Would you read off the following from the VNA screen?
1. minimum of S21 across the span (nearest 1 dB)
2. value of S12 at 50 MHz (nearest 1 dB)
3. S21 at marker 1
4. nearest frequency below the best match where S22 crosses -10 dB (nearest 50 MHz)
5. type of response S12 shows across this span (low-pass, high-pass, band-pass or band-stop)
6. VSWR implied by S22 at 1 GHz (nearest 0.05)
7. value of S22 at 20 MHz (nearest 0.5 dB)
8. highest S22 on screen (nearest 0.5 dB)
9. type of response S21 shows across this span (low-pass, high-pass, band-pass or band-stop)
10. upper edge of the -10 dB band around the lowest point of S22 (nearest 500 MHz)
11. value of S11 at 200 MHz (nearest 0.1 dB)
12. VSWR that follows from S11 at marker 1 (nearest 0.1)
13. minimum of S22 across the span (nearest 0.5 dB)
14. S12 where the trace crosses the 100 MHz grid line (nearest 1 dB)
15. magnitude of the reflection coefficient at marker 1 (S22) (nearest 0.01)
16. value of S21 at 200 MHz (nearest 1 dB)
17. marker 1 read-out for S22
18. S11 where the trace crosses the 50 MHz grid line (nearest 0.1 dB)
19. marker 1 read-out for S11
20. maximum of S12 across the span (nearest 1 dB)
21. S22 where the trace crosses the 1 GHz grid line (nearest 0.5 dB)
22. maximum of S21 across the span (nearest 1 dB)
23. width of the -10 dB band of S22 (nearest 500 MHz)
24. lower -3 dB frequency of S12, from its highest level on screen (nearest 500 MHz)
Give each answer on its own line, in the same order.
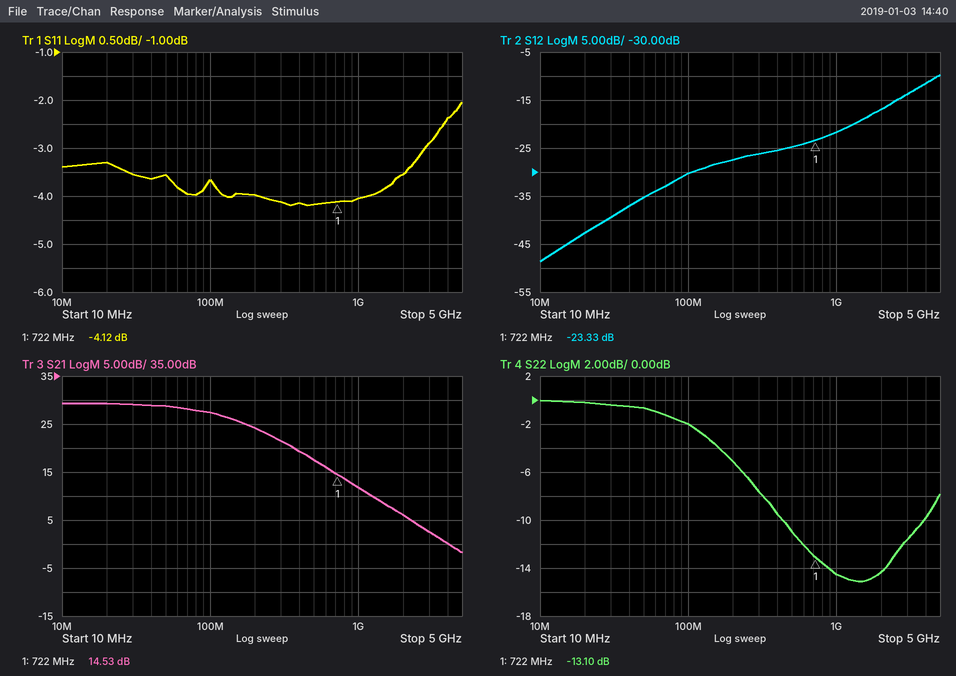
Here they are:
-2 dB
-35 dB
14.53 dB
450 MHz
high-pass
1.45
0.0 dB
0.0 dB
low-pass
4.0 GHz
-4.0 dB
4.3
-15.0 dB
-30 dB
0.22
24 dB
-13.10 dB
-3.6 dB
-4.12 dB
-10 dB
-14.5 dB
29 dB
3.5 GHz
3.5 GHz
